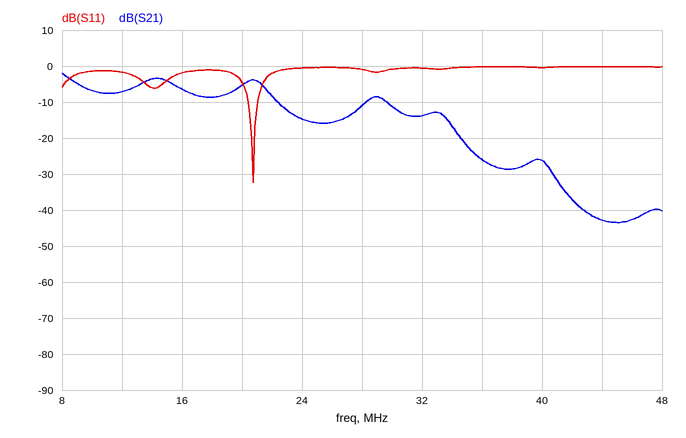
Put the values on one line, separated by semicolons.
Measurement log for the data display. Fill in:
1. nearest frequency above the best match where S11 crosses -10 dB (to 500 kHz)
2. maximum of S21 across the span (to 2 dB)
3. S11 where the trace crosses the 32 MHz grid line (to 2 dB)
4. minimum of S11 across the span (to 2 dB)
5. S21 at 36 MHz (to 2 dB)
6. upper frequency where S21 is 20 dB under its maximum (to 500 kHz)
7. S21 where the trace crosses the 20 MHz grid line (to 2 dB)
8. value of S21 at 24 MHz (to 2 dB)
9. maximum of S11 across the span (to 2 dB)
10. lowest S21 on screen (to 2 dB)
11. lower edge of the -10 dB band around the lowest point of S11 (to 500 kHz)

21.0 MHz; -2 dB; 0 dB; -32 dB; -26 dB; 35.0 MHz; -6 dB; -14 dB; 0 dB; -44 dB; 20.5 MHz
